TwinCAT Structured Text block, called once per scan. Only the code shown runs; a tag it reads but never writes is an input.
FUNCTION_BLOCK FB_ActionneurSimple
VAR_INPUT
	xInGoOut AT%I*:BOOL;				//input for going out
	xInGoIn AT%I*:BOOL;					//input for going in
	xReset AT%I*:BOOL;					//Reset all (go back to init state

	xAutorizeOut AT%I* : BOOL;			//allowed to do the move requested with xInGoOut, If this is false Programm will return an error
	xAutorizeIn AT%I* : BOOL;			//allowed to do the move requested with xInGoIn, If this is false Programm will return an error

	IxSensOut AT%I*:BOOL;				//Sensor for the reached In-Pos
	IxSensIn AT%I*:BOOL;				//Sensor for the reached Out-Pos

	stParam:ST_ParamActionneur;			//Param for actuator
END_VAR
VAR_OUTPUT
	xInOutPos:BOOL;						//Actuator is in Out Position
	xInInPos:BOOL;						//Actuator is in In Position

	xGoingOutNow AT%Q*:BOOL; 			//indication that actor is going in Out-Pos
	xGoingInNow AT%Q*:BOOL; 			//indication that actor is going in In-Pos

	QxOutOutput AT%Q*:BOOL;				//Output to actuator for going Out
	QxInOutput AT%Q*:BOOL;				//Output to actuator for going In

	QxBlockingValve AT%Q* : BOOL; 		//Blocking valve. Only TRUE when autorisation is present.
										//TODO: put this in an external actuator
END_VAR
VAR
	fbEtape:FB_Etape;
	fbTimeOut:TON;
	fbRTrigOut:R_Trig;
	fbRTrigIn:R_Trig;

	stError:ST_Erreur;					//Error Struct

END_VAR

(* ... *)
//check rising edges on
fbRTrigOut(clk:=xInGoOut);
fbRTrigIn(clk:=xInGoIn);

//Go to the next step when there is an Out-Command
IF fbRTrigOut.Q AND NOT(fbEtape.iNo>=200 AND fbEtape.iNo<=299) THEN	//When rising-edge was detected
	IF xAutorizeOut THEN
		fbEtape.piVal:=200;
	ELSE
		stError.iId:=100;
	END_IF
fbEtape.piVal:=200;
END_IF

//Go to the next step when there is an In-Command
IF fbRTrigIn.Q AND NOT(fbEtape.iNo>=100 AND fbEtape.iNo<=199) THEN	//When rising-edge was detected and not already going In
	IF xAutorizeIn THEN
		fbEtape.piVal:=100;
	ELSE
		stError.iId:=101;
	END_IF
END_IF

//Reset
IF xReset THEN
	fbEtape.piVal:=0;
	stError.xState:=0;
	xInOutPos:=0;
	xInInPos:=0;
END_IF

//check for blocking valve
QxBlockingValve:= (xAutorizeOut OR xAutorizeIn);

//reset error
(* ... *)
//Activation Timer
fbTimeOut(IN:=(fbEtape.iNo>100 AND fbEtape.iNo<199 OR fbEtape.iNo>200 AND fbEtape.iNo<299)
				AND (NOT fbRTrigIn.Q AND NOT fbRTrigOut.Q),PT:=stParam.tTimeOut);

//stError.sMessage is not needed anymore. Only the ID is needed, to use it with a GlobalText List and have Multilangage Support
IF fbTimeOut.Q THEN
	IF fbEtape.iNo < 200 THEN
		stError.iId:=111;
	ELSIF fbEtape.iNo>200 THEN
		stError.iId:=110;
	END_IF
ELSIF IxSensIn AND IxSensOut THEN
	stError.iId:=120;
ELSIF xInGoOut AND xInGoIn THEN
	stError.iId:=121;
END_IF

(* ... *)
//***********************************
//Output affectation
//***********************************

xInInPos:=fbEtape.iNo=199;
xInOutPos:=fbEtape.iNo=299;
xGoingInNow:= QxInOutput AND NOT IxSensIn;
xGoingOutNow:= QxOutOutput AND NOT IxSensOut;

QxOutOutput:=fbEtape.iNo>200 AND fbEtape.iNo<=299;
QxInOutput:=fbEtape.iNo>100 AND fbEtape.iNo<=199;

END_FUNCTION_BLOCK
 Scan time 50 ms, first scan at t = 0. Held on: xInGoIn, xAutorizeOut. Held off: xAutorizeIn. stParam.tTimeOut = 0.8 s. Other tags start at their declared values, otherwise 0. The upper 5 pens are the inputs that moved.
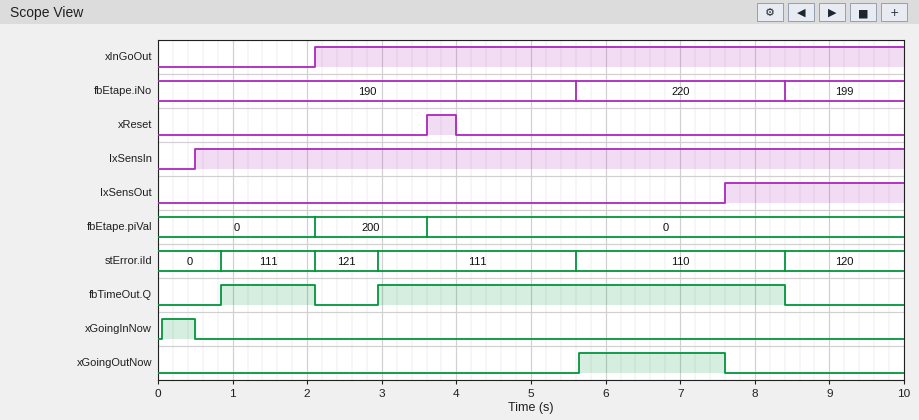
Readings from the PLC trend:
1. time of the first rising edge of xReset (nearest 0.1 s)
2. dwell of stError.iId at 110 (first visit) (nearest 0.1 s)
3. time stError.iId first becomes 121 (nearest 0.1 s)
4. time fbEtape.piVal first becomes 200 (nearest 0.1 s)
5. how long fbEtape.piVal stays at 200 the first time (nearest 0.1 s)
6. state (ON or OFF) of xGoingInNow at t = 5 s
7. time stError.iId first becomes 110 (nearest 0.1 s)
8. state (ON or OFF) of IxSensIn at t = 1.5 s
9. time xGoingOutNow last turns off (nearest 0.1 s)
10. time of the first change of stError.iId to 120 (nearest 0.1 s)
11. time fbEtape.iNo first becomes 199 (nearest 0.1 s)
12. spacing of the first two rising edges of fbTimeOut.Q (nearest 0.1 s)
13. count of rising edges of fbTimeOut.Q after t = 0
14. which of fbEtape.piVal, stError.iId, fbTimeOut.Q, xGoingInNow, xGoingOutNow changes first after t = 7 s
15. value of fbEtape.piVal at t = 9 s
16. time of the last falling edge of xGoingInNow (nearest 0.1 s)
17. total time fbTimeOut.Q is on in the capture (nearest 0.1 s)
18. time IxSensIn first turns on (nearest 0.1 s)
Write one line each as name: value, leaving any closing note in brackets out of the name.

time of the first rising edge of xReset: 3.6 s
dwell of stError.iId at 110 (first visit): 2.8 s
time stError.iId first becomes 121: 2.1 s
time fbEtape.piVal first becomes 200: 2.1 s
how long fbEtape.piVal stays at 200 the first time: 1.5 s
state (ON or OFF) of xGoingInNow at t = 5 s: OFF
time stError.iId first becomes 110: 5.6 s
state (ON or OFF) of IxSensIn at t = 1.5 s: ON
time xGoingOutNow last turns off: 7.6 s
time of the first change of stError.iId to 120: 8.4 s
time fbEtape.iNo first becomes 199: 8.4 s
spacing of the first two rising edges of fbTimeOut.Q: 2.1 s
count of rising edges of fbTimeOut.Q after t = 0: 2
which of fbEtape.piVal, stError.iId, fbTimeOut.Q, xGoingInNow, xGoingOutNow changes first after t = 7 s: xGoingOutNow
value of fbEtape.piVal at t = 9 s: 0
time of the last falling edge of xGoingInNow: 0.5 s
total time fbTimeOut.Q is on in the capture: 6.7 s
time IxSensIn first turns on: 0.5 s
